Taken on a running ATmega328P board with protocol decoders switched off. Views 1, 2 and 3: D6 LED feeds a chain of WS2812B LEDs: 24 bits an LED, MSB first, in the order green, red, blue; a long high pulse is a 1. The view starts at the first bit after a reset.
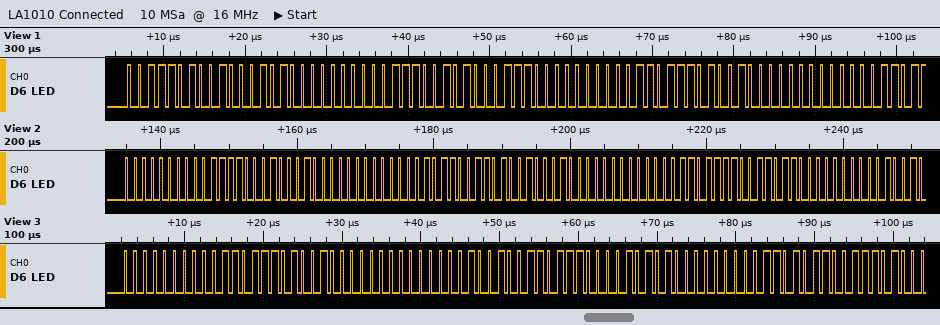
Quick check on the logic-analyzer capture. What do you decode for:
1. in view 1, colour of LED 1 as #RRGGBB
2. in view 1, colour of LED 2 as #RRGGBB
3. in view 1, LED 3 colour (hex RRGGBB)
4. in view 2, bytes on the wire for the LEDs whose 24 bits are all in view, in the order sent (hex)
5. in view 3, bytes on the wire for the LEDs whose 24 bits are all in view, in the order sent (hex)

#453A00
#473900
#483700
00 3C 44 00 16 69 10 00 6F
00 37 48 00 12 6E 15 00 6B
